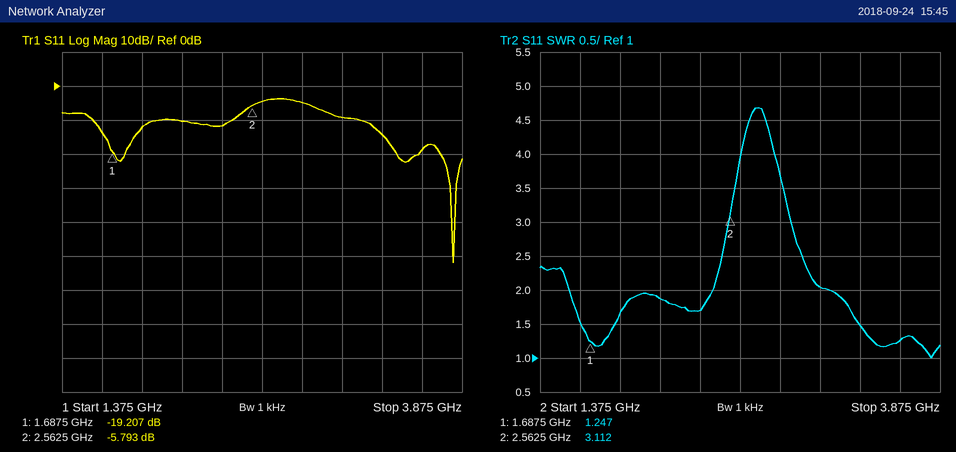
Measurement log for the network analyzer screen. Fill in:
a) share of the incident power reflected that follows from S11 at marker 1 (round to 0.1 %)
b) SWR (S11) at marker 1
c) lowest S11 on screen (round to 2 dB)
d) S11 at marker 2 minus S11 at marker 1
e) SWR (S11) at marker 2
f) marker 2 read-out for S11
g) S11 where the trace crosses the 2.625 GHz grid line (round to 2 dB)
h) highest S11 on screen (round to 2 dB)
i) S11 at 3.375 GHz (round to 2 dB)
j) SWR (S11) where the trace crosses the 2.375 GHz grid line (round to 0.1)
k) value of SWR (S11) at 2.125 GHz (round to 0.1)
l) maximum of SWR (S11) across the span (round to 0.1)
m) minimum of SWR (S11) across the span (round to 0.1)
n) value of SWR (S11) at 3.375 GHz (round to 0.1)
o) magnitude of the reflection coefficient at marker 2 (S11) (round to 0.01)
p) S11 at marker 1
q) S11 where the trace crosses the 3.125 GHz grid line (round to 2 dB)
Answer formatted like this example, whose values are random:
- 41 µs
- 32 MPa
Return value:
- 1.2 %
- 1.247
- -52 dB
- 13.414 dB
- 3.112
- -5.793 dB
- -4 dB
- -4 dB
- -14 dB
- 1.7
- 1.9
- 4.7
- 1.0
- 1.5
- 0.51
- -19.207 dB
- -10 dB
